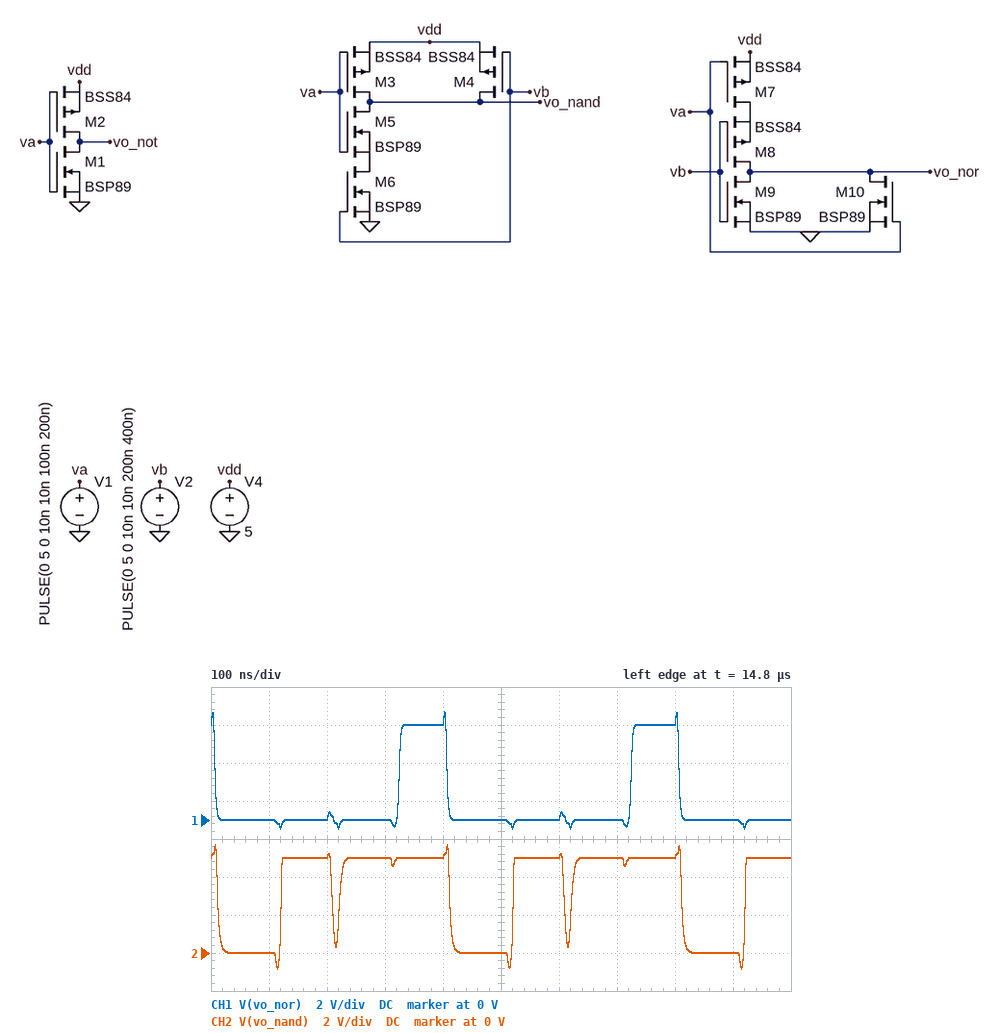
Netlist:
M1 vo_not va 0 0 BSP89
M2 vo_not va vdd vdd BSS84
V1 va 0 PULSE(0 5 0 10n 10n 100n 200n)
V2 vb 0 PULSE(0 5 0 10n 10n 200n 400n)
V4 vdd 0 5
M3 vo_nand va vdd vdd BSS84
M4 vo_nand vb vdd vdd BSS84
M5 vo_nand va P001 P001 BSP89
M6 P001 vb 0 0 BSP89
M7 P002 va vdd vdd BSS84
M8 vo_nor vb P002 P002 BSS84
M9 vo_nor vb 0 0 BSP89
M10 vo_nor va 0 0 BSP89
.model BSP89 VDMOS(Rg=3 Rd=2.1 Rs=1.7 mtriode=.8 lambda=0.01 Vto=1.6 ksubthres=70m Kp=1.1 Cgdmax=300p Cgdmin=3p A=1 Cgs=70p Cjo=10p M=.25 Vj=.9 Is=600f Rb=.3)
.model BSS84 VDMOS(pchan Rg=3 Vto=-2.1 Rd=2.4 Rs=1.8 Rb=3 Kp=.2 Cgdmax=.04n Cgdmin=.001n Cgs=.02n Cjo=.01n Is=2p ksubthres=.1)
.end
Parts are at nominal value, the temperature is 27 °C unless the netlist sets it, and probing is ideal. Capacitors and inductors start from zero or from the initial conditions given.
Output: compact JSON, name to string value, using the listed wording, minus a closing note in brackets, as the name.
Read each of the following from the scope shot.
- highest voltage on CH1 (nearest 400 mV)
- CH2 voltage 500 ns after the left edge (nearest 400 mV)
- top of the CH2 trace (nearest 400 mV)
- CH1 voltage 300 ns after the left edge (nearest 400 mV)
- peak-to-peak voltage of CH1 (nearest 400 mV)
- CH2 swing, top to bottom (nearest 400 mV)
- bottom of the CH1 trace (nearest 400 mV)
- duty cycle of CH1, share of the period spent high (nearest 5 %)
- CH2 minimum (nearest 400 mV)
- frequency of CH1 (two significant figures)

{"highest voltage on CH1": "5.6 V", "CH2 voltage 500 ns after the left edge": "0 V", "top of the CH2 trace": "5.6 V", "CH1 voltage 300 ns after the left edge": "0 V", "peak-to-peak voltage of CH1": "6.0 V", "CH2 swing, top to bottom": "6.4 V", "bottom of the CH1 trace": "-400 mV", "duty cycle of CH1, share of the period spent high": "20 %", "CH2 minimum": "-800 mV", "frequency of CH1": "2.5 MHz"}
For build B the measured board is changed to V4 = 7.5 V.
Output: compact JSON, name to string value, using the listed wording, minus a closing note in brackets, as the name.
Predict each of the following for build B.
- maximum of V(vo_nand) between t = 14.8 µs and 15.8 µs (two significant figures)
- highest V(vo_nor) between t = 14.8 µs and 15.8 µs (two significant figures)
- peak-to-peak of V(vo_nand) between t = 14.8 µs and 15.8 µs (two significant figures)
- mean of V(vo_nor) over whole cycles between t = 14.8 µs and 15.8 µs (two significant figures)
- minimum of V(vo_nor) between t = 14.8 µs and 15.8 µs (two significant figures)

{"maximum of V(vo_nand) between t = 14.8 µs and 15.8 µs": "7.6 V", "highest V(vo_nor) between t = 14.8 µs and 15.8 µs": "8.0 V", "peak-to-peak of V(vo_nand) between t = 14.8 µs and 15.8 µs": "7.5 V", "mean of V(vo_nor) over whole cycles between t = 14.8 µs and 15.8 µs": "1.7 V", "minimum of V(vo_nor) between t = 14.8 µs and 15.8 µs": "-430 mV"}
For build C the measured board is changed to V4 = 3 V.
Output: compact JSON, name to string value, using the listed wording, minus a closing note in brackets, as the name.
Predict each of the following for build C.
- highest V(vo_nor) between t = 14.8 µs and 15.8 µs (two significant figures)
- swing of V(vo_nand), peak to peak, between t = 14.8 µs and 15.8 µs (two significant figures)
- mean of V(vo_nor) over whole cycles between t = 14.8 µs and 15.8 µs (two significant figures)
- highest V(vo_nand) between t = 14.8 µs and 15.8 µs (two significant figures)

{"highest V(vo_nor) between t = 14.8 µs and 15.8 µs": "4.3 V", "swing of V(vo_nand), peak to peak, between t = 14.8 µs and 15.8 µs": "4.9 V", "mean of V(vo_nor) over whole cycles between t = 14.8 µs and 15.8 µs": "430 mV", "highest V(vo_nand) between t = 14.8 µs and 15.8 µs": "3.7 V"}
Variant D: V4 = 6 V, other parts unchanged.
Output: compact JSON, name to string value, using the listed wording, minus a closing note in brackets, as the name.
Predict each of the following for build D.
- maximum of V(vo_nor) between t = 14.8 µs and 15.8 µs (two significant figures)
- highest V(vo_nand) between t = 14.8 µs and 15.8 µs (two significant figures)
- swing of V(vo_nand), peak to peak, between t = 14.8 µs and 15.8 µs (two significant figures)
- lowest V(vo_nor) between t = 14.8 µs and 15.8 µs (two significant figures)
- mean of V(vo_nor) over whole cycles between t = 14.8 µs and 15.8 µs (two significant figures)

{"maximum of V(vo_nor) between t = 14.8 µs and 15.8 µs": "6.6 V", "highest V(vo_nand) between t = 14.8 µs and 15.8 µs": "6.3 V", "swing of V(vo_nand), peak to peak, between t = 14.8 µs and 15.8 µs": "6.9 V", "lowest V(vo_nor) between t = 14.8 µs and 15.8 µs": "-460 mV", "mean of V(vo_nor) over whole cycles between t = 14.8 µs and 15.8 µs": "1.3 V"}
